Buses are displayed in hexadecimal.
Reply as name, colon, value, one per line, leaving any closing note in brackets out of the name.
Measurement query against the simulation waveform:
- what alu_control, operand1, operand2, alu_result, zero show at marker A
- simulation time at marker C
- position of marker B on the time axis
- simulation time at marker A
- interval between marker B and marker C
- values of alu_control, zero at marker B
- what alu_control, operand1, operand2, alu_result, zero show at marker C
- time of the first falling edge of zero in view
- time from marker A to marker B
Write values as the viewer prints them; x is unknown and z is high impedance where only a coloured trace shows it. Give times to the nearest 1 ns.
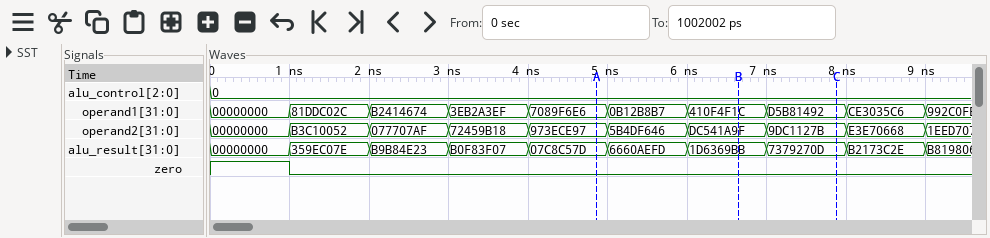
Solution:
what alu_control, operand1, operand2, alu_result, zero show at marker A: alu_control=0, operand1=7089F6E6, operand2=973ECE97, alu_result=07C8C57D, zero=0
simulation time at marker C: 8 ns
position of marker B on the time axis: 7 ns
simulation time at marker A: 5 ns
interval between marker B and marker C: 1 ns
values of alu_control, zero at marker B: alu_control=0, zero=0
what alu_control, operand1, operand2, alu_result, zero show at marker C: alu_control=0, operand1=D5B81492, operand2=9DC1127B, alu_result=7379270D, zero=0
time of the first falling edge of zero in view: 1 ns
time from marker A to marker B: 2 ns
